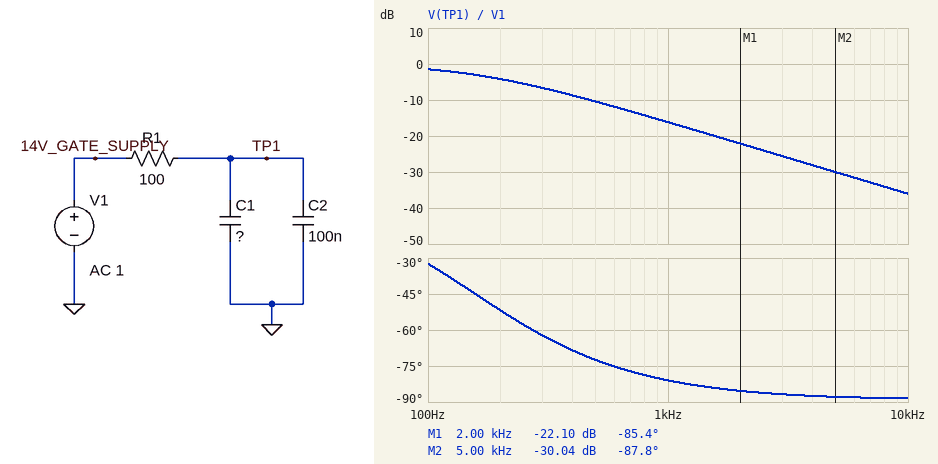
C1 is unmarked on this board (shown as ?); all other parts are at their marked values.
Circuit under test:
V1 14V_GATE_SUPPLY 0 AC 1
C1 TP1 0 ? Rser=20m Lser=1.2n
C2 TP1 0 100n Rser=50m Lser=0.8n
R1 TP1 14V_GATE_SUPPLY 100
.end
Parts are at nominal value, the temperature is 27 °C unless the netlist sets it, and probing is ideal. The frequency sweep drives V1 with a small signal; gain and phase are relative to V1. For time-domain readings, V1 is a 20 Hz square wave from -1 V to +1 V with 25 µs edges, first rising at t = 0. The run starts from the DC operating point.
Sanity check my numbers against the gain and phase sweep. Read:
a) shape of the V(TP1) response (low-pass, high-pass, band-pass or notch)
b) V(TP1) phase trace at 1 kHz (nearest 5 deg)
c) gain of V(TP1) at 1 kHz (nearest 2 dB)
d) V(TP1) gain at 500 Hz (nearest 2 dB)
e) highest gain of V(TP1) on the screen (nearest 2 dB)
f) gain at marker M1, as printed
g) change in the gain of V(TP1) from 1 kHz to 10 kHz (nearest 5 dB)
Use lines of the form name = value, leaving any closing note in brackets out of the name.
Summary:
shape of the V(TP1) response = low-pass
V(TP1) phase trace at 1 kHz = -80 deg
gain of V(TP1) at 1 kHz = -16 dB
V(TP1) gain at 500 Hz = -10 dB
highest gain of V(TP1) on the screen = -2 dB
gain at marker M1, as printed = -22.10 dB
change in the gain of V(TP1) from 1 kHz to 10 kHz = -20 dB
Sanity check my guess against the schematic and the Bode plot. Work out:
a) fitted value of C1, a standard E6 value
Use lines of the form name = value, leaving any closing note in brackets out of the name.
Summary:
fitted value of C1, a standard E6 value = 10 µF
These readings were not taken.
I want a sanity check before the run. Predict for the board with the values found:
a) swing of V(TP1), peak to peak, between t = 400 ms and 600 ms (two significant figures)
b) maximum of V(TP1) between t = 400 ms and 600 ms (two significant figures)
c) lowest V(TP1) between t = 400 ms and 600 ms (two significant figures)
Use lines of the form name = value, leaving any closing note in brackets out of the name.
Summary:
swing of V(TP1), peak to peak, between t = 400 ms and 600 ms = 2.0 V
maximum of V(TP1) between t = 400 ms and 600 ms = 1.0 V
lowest V(TP1) between t = 400 ms and 600 ms = -1.0 V
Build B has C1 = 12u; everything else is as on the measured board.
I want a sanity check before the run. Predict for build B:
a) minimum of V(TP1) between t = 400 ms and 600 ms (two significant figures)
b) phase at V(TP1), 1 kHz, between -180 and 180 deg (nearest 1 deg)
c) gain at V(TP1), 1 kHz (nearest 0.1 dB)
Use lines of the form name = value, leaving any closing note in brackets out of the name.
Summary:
minimum of V(TP1) between t = 400 ms and 600 ms = -1.0 V
phase at V(TP1), 1 kHz, between -180 and 180 deg = -82 deg
gain at V(TP1), 1 kHz = -17.7 dB
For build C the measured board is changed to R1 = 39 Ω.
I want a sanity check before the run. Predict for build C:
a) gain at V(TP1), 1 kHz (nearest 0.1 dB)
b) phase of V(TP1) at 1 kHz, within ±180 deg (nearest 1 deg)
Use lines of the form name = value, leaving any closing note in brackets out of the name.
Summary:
gain at V(TP1), 1 kHz = -8.5 dB
phase of V(TP1) at 1 kHz, within ±180 deg = -68 deg
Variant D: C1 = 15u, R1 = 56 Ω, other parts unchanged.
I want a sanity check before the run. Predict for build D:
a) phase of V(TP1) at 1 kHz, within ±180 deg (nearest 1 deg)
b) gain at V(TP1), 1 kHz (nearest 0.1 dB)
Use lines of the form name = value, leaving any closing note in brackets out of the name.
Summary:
phase of V(TP1) at 1 kHz, within ±180 deg = -79 deg
gain at V(TP1), 1 kHz = -14.7 dB
